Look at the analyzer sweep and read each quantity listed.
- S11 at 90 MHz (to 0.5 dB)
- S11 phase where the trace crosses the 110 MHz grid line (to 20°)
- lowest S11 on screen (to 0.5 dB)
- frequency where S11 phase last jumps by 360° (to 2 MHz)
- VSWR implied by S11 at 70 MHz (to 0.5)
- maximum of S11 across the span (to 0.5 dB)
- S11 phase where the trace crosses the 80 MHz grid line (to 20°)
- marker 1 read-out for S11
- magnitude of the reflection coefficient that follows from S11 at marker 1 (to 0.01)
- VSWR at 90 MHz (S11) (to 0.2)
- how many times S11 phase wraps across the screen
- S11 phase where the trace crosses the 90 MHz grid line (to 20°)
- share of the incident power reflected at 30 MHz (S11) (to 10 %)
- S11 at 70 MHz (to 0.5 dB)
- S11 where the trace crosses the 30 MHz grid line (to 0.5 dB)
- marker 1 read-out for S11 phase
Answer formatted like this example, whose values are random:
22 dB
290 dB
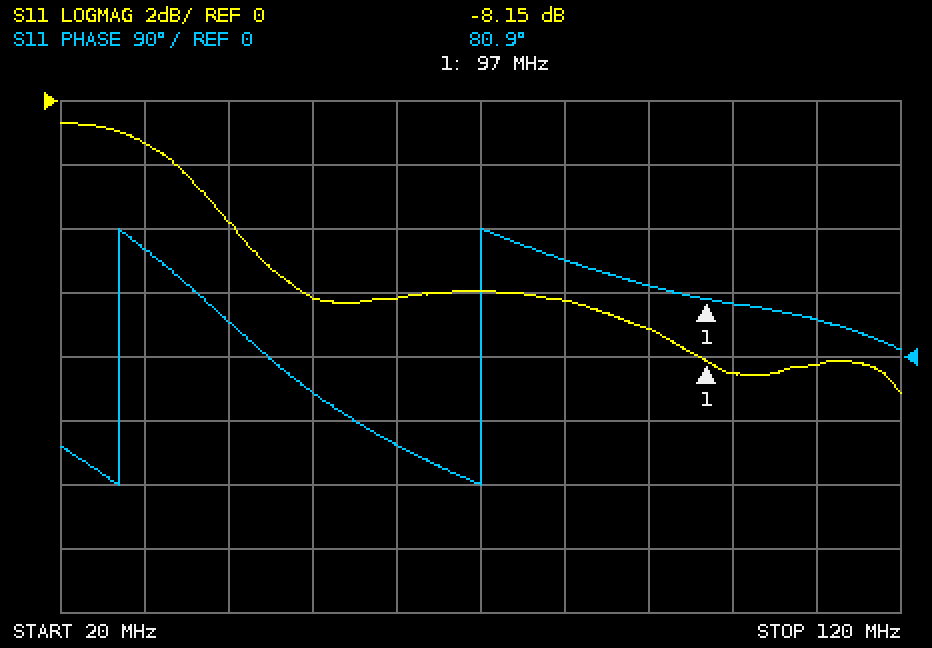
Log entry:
-7.0 dB
60°
-9.0 dB
70 MHz
3.0
-0.5 dB
140°
-8.15 dB
0.39
2.6
2
100°
70 %
-6.0 dB
-1.5 dB
80.9°
